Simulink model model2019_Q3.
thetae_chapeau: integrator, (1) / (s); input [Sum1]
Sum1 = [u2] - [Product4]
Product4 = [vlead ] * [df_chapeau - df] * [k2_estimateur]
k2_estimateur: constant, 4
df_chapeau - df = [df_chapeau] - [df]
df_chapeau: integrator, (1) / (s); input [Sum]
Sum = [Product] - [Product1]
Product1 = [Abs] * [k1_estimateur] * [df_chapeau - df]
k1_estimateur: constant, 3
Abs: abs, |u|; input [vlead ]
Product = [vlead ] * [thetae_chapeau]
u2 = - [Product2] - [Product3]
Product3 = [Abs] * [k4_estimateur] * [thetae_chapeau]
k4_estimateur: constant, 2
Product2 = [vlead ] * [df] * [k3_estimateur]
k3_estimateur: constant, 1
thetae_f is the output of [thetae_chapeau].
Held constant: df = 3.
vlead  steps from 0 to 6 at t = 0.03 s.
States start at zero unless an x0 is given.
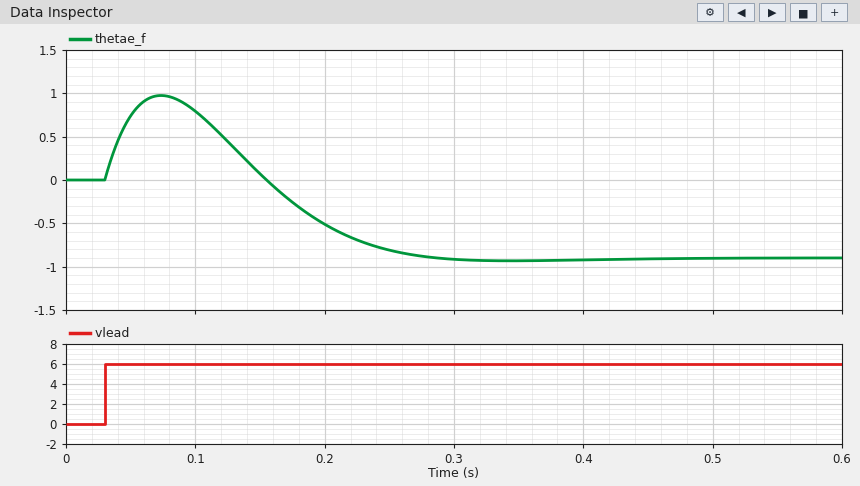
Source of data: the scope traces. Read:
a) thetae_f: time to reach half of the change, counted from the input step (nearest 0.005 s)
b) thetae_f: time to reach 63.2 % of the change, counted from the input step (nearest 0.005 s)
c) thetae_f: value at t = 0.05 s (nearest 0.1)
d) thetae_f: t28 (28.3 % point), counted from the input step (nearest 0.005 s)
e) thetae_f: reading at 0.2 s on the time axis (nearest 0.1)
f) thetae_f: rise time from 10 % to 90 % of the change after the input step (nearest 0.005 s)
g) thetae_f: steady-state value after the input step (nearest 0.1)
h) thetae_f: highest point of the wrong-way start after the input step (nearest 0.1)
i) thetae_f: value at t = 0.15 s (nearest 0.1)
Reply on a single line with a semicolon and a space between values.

0.165 s; 0.175 s; 0.7; 0.145 s; -0.5; 0.090 s; -0.9; 1.0; 0.1
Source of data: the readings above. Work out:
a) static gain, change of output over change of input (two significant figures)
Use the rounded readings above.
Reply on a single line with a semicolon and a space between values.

-0.15
